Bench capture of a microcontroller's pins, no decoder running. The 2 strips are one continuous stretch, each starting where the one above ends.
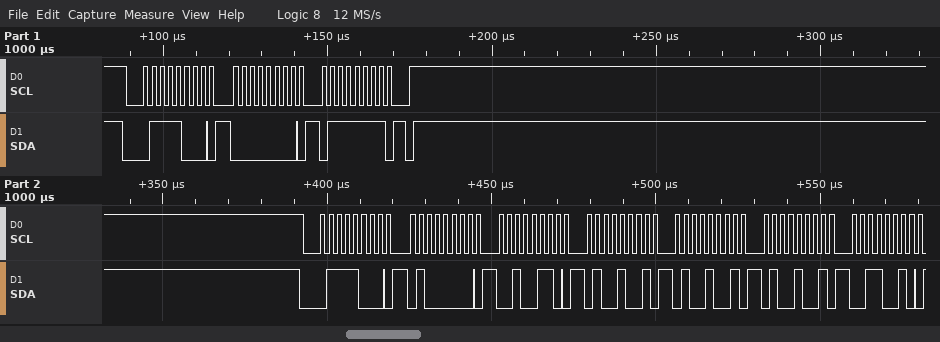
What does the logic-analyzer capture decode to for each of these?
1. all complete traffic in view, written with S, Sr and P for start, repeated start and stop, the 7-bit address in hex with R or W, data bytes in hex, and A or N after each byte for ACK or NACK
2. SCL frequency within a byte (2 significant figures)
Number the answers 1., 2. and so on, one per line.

1. S 3CW A 00 A 7F A P S 3CW A 40 A 26 A 49 A 49 A 49 A 32 A
2. 400 kHz
